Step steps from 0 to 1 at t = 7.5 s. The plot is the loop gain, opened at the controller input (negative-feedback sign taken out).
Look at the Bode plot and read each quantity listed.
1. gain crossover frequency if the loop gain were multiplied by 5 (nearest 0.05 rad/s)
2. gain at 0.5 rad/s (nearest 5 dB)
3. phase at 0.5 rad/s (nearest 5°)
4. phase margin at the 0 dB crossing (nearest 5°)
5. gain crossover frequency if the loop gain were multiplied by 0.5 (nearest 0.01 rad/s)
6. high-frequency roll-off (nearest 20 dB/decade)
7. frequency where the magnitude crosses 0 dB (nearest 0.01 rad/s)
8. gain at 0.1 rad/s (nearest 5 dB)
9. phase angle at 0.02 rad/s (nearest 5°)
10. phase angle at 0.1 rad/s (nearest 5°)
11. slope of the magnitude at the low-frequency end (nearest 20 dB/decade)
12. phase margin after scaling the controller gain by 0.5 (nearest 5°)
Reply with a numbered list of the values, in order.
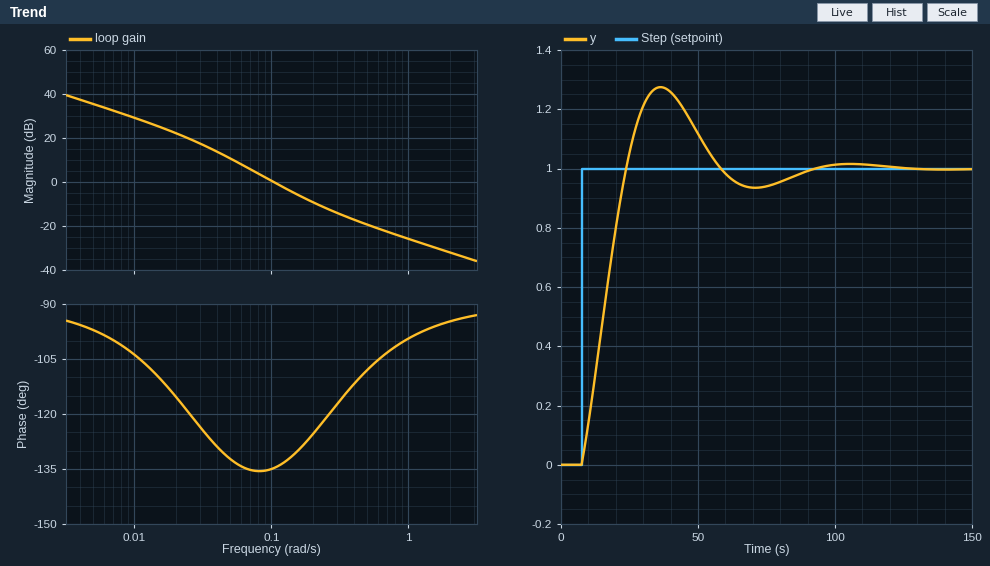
1. 0.30 rad/s
2. -20 dB
3. -110°
4. 45°
5. 0.07 rad/s
6. -20 dB/decade
7. 0.10 rad/s
8. 0 dB
9. -115°
10. -135°
11. -20 dB/decade
12. 45°
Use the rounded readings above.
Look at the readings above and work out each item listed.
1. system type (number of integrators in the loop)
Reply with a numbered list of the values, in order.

1. 1
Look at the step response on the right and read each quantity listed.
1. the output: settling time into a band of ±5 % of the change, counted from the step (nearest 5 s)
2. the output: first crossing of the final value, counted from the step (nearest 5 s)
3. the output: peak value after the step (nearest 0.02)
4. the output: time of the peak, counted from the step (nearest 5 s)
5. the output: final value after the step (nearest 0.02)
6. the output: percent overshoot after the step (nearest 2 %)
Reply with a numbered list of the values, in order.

1. 70 s
2. 15 s
3. 1.28
4. 30 s
5. 1.00
6. 28 %
